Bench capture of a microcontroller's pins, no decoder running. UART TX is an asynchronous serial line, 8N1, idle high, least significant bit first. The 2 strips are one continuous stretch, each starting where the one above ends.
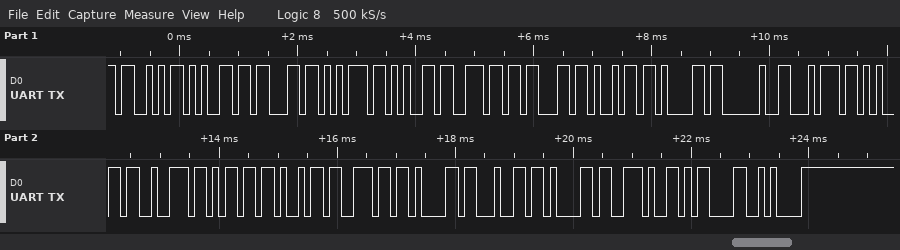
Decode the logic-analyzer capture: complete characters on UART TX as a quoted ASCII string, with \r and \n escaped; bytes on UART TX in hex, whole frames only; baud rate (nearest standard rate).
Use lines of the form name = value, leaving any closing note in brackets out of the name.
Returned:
complete characters on UART TX as a quoted ASCII string, with \r and \n escaped = "Secuencia terminada.\r\n"
bytes on UART TX in hex, whole frames only = 53 65 63 75 65 6E 63 69 61 20 74 65 72 6D 69 6E 61 64 61 2E 0D 0A
baud rate = 9600 baud
